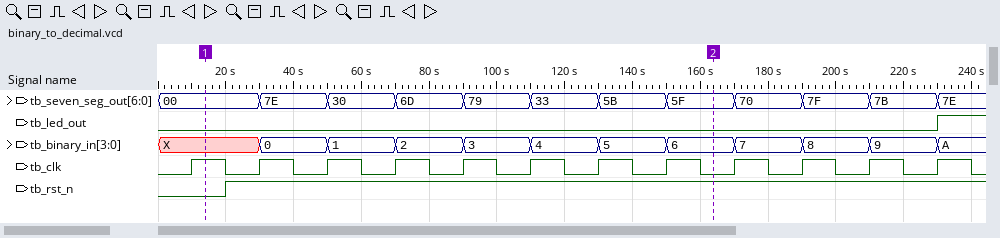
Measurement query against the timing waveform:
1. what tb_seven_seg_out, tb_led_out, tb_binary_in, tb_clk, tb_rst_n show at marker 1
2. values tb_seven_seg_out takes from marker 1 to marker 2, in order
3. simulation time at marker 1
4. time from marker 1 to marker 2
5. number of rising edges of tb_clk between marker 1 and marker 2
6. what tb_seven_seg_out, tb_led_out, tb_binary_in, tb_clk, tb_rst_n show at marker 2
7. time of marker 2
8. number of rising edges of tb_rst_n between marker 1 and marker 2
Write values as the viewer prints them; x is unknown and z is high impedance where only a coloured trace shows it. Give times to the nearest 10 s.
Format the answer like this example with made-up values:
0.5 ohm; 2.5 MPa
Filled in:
tb_seven_seg_out=00, tb_led_out=0, tb_binary_in=X, tb_clk=1, tb_rst_n=0; 00, 7E, 30, 6D, 79, 33, 5B, 5F; 10 s; 150 s; 7; tb_seven_seg_out=5F, tb_led_out=0, tb_binary_in=6, tb_clk=0, tb_rst_n=1; 160 s; 1
